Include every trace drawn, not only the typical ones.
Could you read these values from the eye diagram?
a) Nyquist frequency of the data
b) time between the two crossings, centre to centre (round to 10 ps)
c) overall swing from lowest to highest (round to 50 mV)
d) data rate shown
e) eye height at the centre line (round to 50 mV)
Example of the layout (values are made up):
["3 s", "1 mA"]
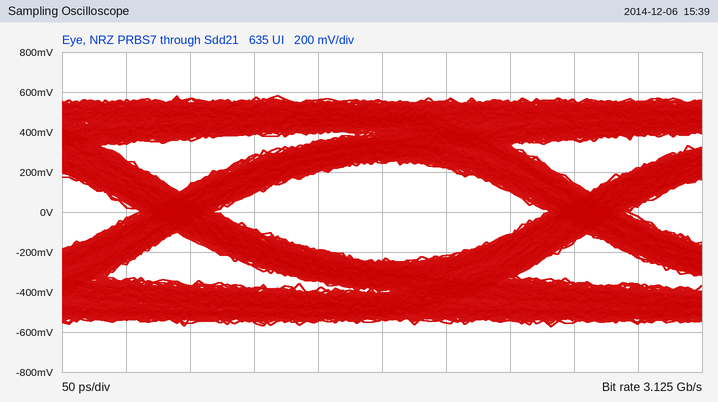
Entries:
["1.5625 GHz", "320 ps", "1.15 V", "3.125 Gb/s", "500 mV"]
